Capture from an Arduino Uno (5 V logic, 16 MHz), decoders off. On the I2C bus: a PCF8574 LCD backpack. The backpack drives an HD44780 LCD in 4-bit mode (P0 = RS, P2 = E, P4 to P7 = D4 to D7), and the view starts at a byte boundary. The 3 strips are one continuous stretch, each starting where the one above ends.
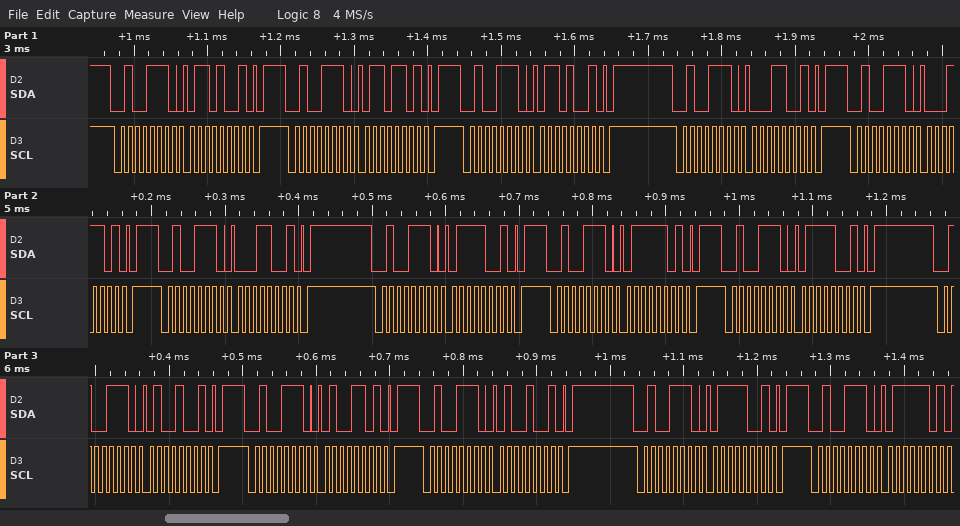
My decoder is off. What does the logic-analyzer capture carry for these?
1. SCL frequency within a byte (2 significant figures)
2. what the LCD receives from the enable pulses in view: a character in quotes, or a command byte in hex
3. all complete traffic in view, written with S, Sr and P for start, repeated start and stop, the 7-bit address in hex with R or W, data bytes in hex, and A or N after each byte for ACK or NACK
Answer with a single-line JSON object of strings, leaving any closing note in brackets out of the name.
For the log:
{"SCL frequency within a byte": "100 kHz", "what the LCD receives from the enable pulses in view: a character in quotes, or a command byte in hex": "'a' 't'", "all complete traffic in view, written with S, Sr and P for start, repeated start and stop, the 7-bit address in hex with R or W, data bytes in hex, and A or N after each byte for ACK or NACK": "S 27W A 69 A P S 27W A 6D A P S 27W A 69 A P S 27W A 19 A P S 27W A 1D A P S 27W A 19 A P S 27W A 79 A P S 27W A 7D A P S 27W A 79 A P S 27W A 49 A P S 27W A 4D A P S 27W A 49 A P S 27W A 79 A P S 27W A 7D A"}
